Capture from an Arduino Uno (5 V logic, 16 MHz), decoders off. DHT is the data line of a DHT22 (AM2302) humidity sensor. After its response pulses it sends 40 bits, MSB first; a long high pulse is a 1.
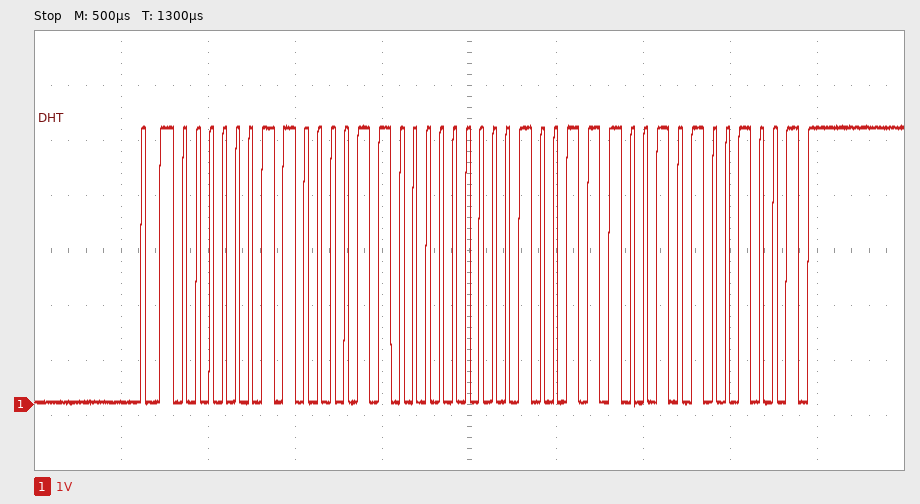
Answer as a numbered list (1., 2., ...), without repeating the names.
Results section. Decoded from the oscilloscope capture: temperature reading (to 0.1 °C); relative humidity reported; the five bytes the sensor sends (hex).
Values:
1. 31.3 °C
2. 78.0 %
3. 03 0C 01 39 49
